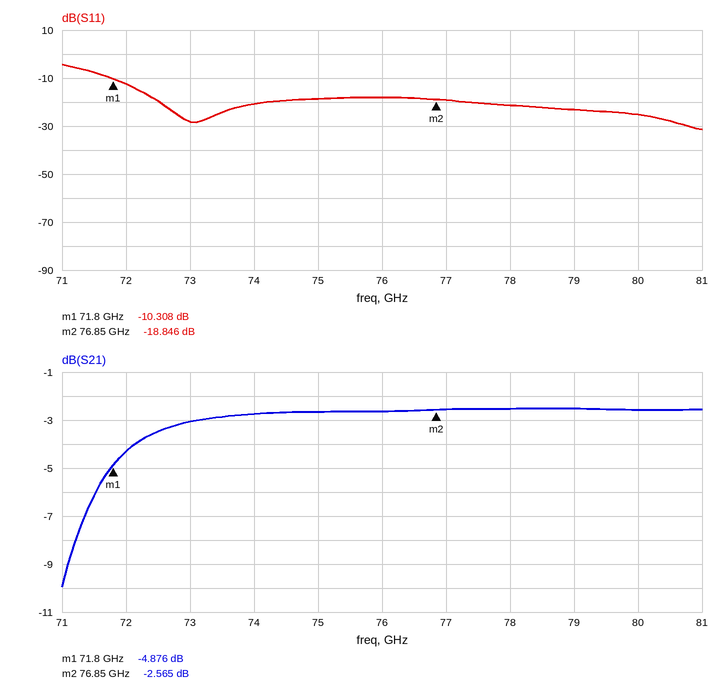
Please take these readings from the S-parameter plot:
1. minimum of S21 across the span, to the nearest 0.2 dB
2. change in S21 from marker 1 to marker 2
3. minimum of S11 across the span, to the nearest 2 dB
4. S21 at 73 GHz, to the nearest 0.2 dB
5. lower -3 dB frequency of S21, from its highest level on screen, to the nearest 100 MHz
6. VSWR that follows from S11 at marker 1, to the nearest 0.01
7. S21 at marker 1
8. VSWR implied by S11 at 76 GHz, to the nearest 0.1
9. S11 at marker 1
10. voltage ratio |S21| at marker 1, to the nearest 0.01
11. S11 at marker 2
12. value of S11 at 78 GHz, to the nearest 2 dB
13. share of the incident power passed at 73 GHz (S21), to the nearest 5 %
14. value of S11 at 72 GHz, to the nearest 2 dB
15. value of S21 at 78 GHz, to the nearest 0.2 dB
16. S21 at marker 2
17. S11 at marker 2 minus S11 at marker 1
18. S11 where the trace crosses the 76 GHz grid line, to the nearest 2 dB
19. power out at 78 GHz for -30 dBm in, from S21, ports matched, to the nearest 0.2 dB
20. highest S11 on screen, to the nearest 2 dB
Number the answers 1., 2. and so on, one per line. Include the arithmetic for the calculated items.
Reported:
1. -10.0 dB
2. -2.565 − (-4.876) = 2.311 dB
3. -32 dB
4. -3.0 dB
5. 71.6 GHz
6. (1 + 0.3052)/(1 − 0.3052) ≈ 1.88
7. -4.876 dB
8. |Γ| = 10^(-18/20) = 0.1259; VSWR = (1 + 0.1259)/(1 − 0.1259) ≈ 1.3
9. -10.308 dB
10. 10^(-4.876/20) ≈ 0.57
11. -18.846 dB
12. -22 dB
13. 10^(-3/10) ≈ 50 %
14. -12 dB
15. -2.6 dB
16. -2.565 dB
17. -18.846 − (-10.308) = -8.538 dB
18. -18 dB
19. -30 dBm + (-2.6 dB) = -32.6 dBm
20. -4 dB
